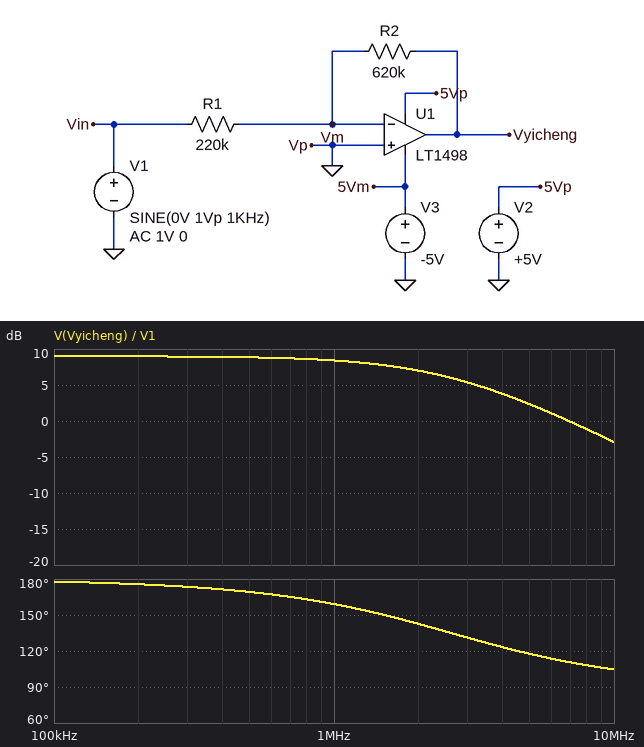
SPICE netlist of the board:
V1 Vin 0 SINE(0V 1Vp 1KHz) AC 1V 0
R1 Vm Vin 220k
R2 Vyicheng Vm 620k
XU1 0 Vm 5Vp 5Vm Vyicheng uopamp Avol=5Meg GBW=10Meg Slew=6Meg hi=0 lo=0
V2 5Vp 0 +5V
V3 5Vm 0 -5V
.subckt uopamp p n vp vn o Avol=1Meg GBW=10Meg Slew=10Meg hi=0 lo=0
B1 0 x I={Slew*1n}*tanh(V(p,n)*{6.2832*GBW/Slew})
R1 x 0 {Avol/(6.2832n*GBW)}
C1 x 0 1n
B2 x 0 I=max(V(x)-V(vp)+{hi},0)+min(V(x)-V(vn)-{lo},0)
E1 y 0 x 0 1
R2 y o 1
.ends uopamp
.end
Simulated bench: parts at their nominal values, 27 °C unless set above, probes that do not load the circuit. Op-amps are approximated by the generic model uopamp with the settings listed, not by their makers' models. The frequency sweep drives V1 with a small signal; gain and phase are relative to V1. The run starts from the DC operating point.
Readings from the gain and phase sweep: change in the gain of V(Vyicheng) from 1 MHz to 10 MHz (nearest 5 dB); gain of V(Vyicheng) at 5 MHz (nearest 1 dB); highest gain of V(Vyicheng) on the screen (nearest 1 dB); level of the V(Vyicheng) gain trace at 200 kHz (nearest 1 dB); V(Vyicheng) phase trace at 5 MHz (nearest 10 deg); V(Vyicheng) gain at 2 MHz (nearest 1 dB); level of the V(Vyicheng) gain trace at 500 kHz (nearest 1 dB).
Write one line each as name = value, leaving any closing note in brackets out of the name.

change in the gain of V(Vyicheng) from 1 MHz to 10 MHz = -10 dB
gain of V(Vyicheng) at 5 MHz = 2 dB
highest gain of V(Vyicheng) on the screen = 9 dB
level of the V(Vyicheng) gain trace at 200 kHz = 9 dB
V(Vyicheng) phase trace at 5 MHz = 120 deg
V(Vyicheng) gain at 2 MHz = 7 dB
level of the V(Vyicheng) gain trace at 500 kHz = 9 dB
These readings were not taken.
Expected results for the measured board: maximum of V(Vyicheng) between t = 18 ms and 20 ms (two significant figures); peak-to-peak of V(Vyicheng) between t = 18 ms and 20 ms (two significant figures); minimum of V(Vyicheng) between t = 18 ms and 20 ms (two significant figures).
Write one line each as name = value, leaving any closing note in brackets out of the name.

maximum of V(Vyicheng) between t = 18 ms and 20 ms = 2.8 V
peak-to-peak of V(Vyicheng) between t = 18 ms and 20 ms = 5.6 V
minimum of V(Vyicheng) between t = 18 ms and 20 ms = -2.8 V
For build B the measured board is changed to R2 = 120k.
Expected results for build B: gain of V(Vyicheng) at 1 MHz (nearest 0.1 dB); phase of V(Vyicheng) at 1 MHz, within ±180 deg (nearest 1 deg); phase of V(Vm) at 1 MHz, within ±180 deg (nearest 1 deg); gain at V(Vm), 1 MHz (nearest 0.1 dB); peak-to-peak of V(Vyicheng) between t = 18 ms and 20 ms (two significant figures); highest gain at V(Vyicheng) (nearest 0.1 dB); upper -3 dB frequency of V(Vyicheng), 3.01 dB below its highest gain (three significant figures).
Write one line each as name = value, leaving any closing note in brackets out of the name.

gain of V(Vyicheng) at 1 MHz = -5.4 dB
phase of V(Vyicheng) at 1 MHz, within ±180 deg = 171 deg
phase of V(Vm) at 1 MHz, within ±180 deg = 81 deg
gain at V(Vm), 1 MHz = -25.4 dB
peak-to-peak of V(Vyicheng) between t = 18 ms and 20 ms = 1.1 V
highest gain at V(Vyicheng) = -5.3 dB
upper -3 dB frequency of V(Vyicheng), 3.01 dB below its highest gain = 6.47 MHz
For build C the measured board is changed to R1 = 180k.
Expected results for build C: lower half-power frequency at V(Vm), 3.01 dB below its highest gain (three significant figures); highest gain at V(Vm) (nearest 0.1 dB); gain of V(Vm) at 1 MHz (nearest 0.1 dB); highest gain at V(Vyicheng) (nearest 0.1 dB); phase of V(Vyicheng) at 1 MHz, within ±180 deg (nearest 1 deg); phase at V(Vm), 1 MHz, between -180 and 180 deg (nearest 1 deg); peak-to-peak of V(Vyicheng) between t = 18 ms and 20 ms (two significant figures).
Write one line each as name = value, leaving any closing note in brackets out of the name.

lower half-power frequency at V(Vm), 3.01 dB below its highest gain = 2.25 MHz
highest gain at V(Vm) = -2.2 dB
gain of V(Vm) at 1 MHz = -10.0 dB
highest gain at V(Vyicheng) = 10.7 dB
phase of V(Vyicheng) at 1 MHz, within ±180 deg = 156 deg
phase at V(Vm), 1 MHz, between -180 and 180 deg = 66 deg
peak-to-peak of V(Vyicheng) between t = 18 ms and 20 ms = 6.9 V
